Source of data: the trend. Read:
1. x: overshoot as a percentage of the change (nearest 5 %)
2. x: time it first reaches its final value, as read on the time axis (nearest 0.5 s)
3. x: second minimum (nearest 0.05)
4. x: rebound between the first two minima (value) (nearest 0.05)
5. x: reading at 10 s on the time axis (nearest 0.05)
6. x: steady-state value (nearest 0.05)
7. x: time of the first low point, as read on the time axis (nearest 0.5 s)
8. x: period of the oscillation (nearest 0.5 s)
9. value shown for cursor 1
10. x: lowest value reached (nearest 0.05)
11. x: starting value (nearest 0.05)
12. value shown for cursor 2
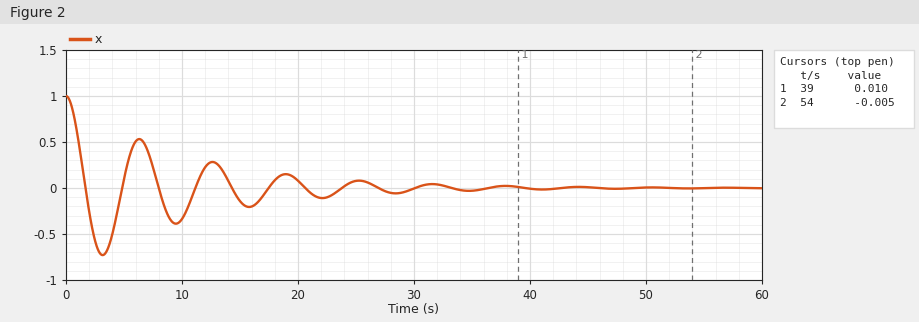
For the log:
75 %
1.5 s
-0.40
0.55
-0.35
0.00
3.0 s
6.5 s
0.010
-0.75
1.00
-0.005
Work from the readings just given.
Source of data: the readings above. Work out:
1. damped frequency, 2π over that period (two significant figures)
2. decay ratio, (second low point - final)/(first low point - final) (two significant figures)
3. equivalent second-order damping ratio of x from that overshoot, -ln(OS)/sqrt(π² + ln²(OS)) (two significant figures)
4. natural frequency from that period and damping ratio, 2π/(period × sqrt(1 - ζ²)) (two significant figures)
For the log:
0.97 rad/s
0.53
0.091
0.97 rad/s
